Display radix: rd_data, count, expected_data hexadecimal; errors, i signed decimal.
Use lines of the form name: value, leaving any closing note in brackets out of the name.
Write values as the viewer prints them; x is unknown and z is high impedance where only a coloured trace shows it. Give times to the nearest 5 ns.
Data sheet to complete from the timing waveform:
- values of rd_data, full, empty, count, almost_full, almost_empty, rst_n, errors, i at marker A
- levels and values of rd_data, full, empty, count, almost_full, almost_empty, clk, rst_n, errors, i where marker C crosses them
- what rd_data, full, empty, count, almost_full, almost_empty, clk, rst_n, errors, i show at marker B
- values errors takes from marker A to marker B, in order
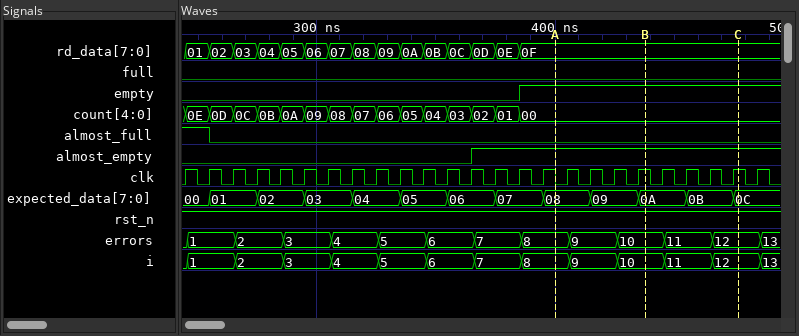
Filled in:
values of rd_data, full, empty, count, almost_full, almost_empty, rst_n, errors, i at marker A: rd_data=0F, full=0, empty=1, count=00, almost_full=0, almost_empty=1, rst_n=1, errors=8, i=8
levels and values of rd_data, full, empty, count, almost_full, almost_empty, clk, rst_n, errors, i where marker C crosses them: rd_data=0F, full=0, empty=1, count=00, almost_full=0, almost_empty=1, clk=1, rst_n=1, errors=12, i=12
what rd_data, full, empty, count, almost_full, almost_empty, clk, rst_n, errors, i show at marker B: rd_data=0F, full=0, empty=1, count=00, almost_full=0, almost_empty=1, clk=1, rst_n=1, errors=10, i=10
values errors takes from marker A to marker B, in order: 8, 9, 10
